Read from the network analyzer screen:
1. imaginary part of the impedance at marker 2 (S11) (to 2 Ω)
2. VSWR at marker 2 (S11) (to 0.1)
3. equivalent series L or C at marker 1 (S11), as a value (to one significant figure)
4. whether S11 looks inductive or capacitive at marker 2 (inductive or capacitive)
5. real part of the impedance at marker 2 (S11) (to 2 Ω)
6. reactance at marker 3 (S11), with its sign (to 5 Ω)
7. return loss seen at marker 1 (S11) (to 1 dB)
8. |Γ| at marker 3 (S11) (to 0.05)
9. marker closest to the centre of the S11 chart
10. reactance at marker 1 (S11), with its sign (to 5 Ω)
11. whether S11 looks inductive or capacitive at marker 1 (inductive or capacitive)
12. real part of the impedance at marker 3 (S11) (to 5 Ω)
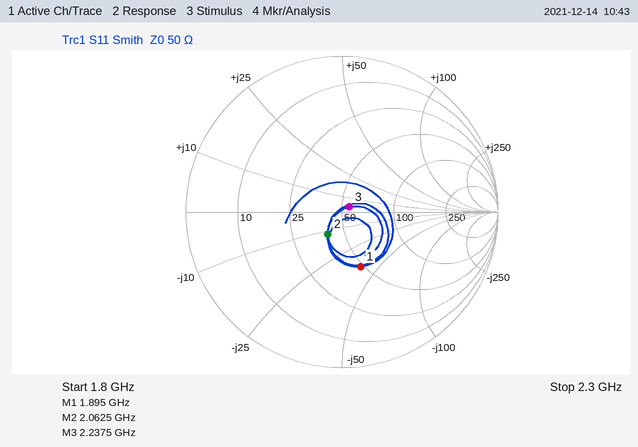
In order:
-12 Ω
1.4
2 pF
capacitive
40 Ω
+5 Ω
9 dB
0.05
marker 3
-40 Ω
capacitive
55 Ω
